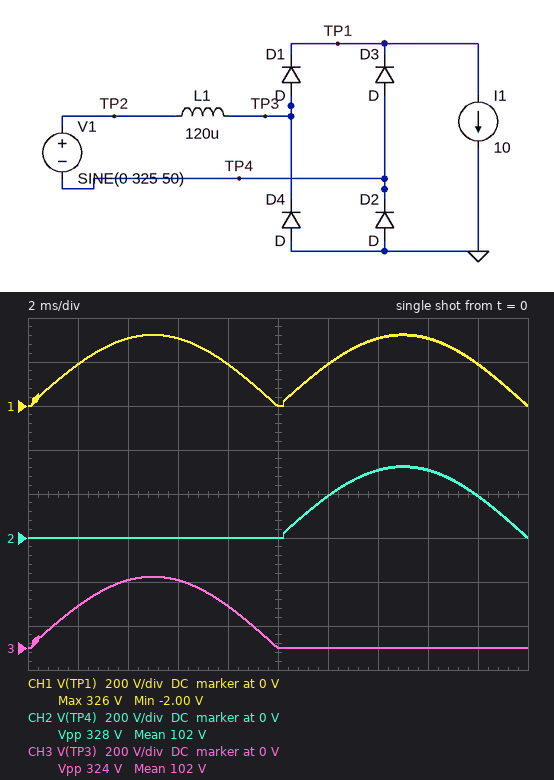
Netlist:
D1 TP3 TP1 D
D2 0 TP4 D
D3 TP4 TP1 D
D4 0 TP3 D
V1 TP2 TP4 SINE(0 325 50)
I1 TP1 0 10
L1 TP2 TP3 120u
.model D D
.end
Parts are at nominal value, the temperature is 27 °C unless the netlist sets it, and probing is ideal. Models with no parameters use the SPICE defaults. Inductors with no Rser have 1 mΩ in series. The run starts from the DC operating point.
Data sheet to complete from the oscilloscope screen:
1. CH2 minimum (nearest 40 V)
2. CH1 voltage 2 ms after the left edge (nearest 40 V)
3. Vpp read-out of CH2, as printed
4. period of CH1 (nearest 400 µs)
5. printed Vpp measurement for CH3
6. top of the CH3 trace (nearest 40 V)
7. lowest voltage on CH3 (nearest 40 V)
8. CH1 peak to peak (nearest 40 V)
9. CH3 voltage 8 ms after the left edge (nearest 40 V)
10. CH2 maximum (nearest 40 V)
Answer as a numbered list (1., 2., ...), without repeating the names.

1. 0 V
2. 200 V
3. 328 V
4. 10.0 ms
5. 324 V
6. 320 V
7. 0 V
8. 320 V
9. 200 V
10. 320 V
